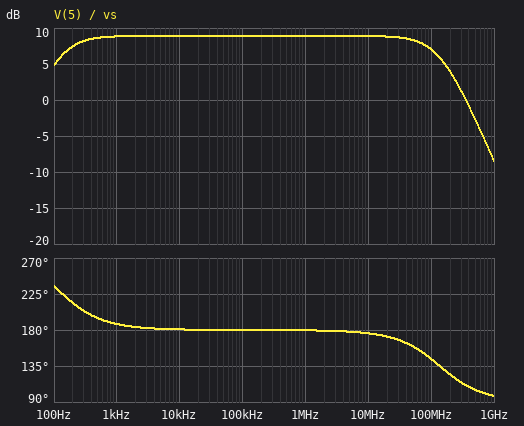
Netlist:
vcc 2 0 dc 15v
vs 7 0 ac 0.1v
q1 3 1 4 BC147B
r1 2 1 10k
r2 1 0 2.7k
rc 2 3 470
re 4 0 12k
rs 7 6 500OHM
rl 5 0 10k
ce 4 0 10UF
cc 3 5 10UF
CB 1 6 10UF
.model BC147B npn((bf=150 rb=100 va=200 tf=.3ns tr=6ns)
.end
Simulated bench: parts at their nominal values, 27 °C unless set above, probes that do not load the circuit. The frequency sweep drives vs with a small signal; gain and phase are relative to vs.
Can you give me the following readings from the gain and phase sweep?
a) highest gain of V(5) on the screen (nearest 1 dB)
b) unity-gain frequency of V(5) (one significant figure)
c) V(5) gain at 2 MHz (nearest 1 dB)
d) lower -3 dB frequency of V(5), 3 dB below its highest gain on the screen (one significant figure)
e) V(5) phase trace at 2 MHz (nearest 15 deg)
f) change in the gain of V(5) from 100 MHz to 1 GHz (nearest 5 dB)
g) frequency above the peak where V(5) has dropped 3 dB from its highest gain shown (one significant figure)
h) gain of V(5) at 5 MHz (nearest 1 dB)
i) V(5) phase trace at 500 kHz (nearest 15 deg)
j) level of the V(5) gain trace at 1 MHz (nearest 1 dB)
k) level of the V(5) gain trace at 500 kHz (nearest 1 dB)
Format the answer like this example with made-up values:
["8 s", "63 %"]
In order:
["9 dB", "400 MHz", "9 dB", "100 Hz", "180 deg", "-15 dB", "100 MHz", "9 dB", "180 deg", "9 dB", "9 dB"]
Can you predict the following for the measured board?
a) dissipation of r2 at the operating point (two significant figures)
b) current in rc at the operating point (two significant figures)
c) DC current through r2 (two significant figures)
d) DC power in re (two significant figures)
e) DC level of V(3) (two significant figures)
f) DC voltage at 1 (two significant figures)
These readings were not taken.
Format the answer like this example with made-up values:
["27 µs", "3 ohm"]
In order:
["3.8 mW", "200 µA", "1.2 mA", "500 µW", "15 V", "3.2 V"]
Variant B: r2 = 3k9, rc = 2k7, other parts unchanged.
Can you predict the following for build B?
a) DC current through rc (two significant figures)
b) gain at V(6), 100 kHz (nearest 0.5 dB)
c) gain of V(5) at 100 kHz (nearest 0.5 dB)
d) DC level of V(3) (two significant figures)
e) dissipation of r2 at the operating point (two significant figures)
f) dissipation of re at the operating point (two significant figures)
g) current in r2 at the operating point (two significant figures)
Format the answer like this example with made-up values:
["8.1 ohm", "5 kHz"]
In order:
["290 µA", "-1.5 dB", "25.5 dB", "14 V", "4.5 mW", "1.0 mW", "1.1 mA"]
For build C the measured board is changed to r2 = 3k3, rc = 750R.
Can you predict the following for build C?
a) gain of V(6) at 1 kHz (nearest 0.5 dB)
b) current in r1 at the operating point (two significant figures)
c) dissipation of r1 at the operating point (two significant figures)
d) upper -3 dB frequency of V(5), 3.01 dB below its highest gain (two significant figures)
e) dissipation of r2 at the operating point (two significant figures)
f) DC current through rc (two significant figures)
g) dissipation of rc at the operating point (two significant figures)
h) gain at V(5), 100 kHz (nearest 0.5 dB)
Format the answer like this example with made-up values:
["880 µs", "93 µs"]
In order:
["-2.0 dB", "1.1 mA", "13 mW", "110 MHz", "4.2 mW", "250 µA", "46 µW", "14.5 dB"]
